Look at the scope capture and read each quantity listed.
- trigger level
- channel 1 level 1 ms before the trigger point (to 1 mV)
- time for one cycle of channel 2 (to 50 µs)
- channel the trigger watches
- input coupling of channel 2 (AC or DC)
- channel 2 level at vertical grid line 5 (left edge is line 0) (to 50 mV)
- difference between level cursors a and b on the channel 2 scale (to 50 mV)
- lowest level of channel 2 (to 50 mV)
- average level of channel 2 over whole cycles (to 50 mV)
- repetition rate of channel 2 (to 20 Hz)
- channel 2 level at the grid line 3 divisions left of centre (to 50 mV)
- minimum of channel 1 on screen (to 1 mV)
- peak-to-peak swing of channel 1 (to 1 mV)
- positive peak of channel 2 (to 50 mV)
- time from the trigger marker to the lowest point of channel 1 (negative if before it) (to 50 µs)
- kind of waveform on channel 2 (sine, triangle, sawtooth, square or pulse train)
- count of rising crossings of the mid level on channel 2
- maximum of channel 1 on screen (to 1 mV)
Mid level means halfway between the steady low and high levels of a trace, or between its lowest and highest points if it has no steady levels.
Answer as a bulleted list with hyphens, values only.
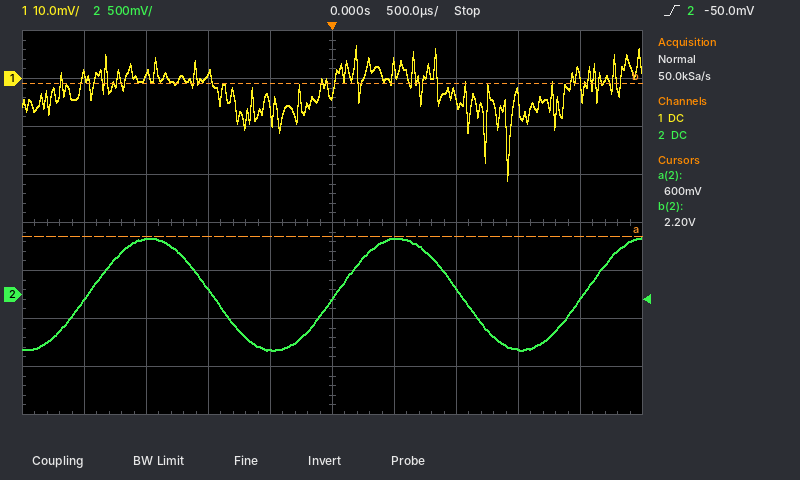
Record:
- -50.0 mV
- 1 mV
- 2.00 ms
- channel 2
- DC
- -50 mV
- 1.60 V
- -600 mV
- 0 mV
- 500 Hz
- 600 mV
- -21 mV
- 28 mV
- 600 mV
- +1.40 ms
- sine
- 3
- 7 mV
